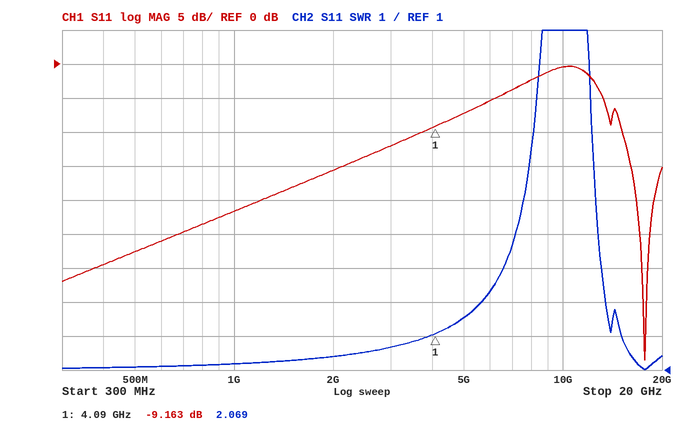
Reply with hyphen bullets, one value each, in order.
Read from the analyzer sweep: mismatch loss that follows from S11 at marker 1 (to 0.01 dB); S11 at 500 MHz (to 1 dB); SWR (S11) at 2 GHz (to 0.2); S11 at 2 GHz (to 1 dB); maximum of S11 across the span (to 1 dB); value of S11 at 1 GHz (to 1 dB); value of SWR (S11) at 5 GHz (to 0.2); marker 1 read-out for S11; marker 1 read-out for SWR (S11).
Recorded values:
- 0.56 dB
- -28 dB
- 1.4
- -16 dB
- 0 dB
- -22 dB
- 2.6
- -9.163 dB
- 2.069
